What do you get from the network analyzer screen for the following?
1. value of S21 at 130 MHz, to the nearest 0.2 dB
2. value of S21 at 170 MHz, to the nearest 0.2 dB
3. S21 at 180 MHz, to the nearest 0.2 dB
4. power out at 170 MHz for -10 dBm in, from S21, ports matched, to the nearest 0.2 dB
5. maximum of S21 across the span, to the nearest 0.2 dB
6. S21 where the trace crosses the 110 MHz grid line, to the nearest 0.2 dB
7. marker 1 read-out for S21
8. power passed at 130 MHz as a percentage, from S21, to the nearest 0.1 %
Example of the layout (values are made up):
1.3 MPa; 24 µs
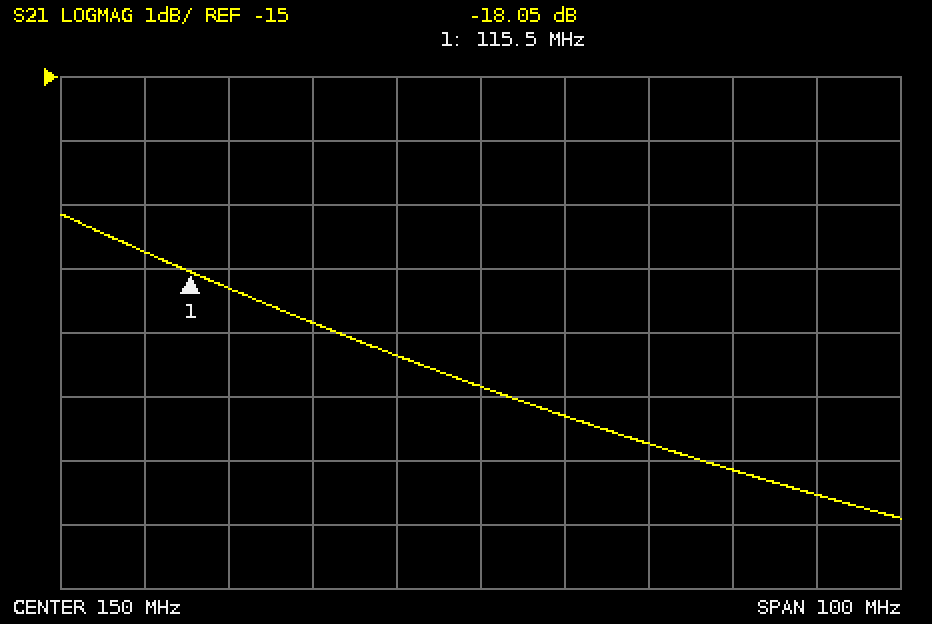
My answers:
-18.8 dB; -20.8 dB; -21.2 dB; -30.8 dBm; -17.2 dB; -17.8 dB; -18.05 dB; 1.3 %
